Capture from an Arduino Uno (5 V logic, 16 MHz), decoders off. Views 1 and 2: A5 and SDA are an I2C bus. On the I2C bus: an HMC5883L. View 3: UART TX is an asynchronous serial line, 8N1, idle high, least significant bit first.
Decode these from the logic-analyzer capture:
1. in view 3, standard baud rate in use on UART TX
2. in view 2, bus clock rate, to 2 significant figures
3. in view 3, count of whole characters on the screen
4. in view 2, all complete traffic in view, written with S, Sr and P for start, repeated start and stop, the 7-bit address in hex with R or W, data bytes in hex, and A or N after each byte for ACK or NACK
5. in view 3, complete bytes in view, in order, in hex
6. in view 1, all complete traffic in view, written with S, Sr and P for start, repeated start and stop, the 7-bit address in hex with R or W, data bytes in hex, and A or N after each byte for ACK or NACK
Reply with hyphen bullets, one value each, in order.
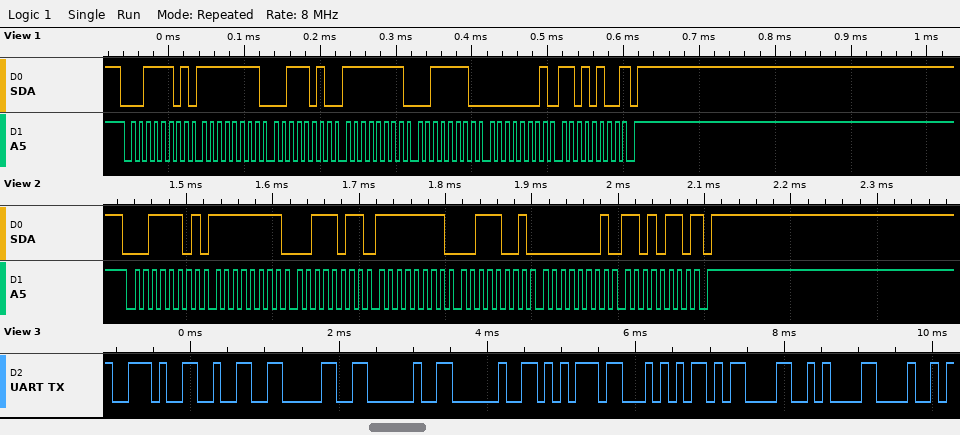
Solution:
- 9600 baud
- 100 kHz
- 10
- S 1ER A FF A 3B A FF A 39 A 01 A D6 N P
- 0x2E 0x32 0x30 0x20 0x20 0x75 0x54 0x0D 0x0A 0x48
- S 1ER A FF A 3A A FF A 3E A 01 A D4 N P
